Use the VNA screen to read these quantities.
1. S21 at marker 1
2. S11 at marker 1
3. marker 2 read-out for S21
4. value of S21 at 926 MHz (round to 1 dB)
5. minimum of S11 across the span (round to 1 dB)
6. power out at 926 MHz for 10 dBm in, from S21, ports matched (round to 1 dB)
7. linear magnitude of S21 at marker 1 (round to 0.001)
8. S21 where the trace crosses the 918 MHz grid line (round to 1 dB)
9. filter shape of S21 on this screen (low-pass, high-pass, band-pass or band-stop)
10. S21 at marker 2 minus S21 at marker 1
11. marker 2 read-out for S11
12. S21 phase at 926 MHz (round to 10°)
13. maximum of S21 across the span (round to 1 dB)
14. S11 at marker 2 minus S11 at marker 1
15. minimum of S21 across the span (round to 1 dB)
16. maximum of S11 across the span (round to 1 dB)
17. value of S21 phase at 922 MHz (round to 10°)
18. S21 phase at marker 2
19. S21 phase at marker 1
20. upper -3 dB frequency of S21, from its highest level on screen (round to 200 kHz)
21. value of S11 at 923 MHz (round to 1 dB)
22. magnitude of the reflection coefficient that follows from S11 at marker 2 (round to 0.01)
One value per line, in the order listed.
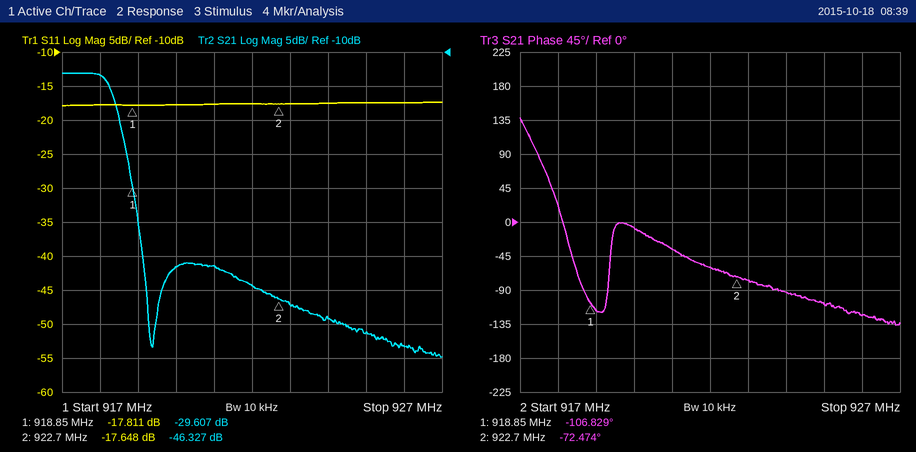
-29.607 dB
-17.811 dB
-46.327 dB
-53 dB
-18 dB
-43 dBm
0.033
-13 dB
low-pass
-16.720 dB
-17.648 dB
-120°
-13 dB
0.163 dB
-55 dB
-17 dB
-60°
-72.474°
-106.829°
918.4 MHz
-18 dB
0.13
